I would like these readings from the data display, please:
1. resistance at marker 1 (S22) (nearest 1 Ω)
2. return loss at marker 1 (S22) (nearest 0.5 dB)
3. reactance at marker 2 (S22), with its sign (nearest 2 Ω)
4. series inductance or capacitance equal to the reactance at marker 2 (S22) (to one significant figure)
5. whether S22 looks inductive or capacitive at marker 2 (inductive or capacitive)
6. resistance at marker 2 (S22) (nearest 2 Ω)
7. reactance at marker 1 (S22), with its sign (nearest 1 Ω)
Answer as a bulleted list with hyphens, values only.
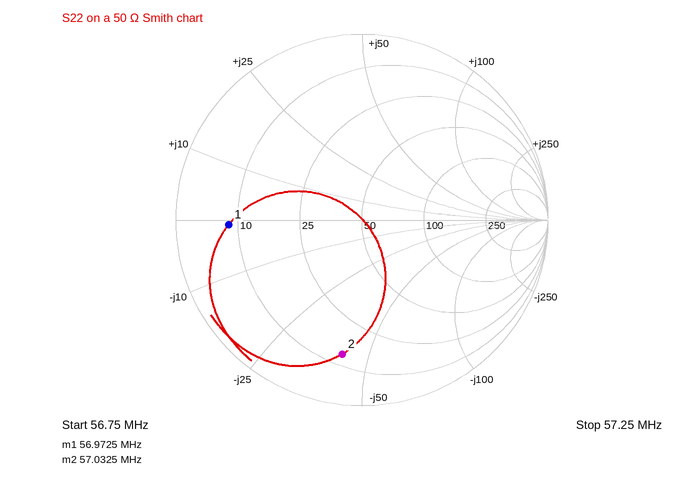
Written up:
- 8 Ω
- 3.0 dB
- -42 Ω
- 70 pF
- capacitive
- 14 Ω
- -1 Ω
